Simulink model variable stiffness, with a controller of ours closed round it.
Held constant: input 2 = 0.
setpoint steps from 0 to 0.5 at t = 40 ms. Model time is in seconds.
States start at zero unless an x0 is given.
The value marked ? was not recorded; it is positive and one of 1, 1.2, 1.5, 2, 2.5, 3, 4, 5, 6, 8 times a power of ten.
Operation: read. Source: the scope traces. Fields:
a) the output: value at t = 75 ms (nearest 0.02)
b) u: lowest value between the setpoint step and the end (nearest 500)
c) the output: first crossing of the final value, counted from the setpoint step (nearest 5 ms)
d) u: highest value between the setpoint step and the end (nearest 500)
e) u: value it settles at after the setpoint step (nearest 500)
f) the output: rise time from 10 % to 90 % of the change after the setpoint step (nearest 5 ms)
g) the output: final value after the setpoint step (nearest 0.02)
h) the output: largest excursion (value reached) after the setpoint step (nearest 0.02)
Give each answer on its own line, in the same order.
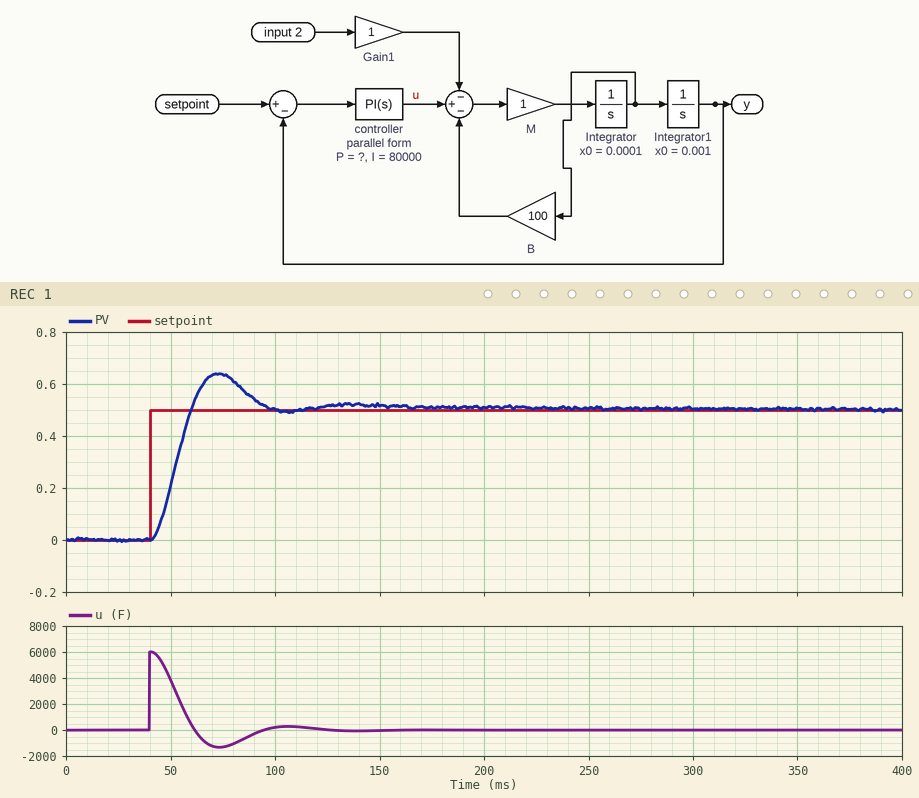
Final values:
0.64
-1500
20 ms
6000
0
15 ms
0.50
0.64
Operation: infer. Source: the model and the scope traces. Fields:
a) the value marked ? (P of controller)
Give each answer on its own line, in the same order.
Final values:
12000
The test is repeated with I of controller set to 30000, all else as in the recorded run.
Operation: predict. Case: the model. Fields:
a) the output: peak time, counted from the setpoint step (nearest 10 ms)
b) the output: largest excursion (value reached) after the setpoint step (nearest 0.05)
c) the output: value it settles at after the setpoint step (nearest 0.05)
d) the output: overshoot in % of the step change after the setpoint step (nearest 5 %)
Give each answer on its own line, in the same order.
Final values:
30 ms
0.60
0.50
25 %
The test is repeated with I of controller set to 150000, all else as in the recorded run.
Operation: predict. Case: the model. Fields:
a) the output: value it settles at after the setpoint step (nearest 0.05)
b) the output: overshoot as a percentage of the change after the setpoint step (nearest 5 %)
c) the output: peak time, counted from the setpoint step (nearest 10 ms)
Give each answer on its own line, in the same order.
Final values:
0.50
35 %
30 ms
